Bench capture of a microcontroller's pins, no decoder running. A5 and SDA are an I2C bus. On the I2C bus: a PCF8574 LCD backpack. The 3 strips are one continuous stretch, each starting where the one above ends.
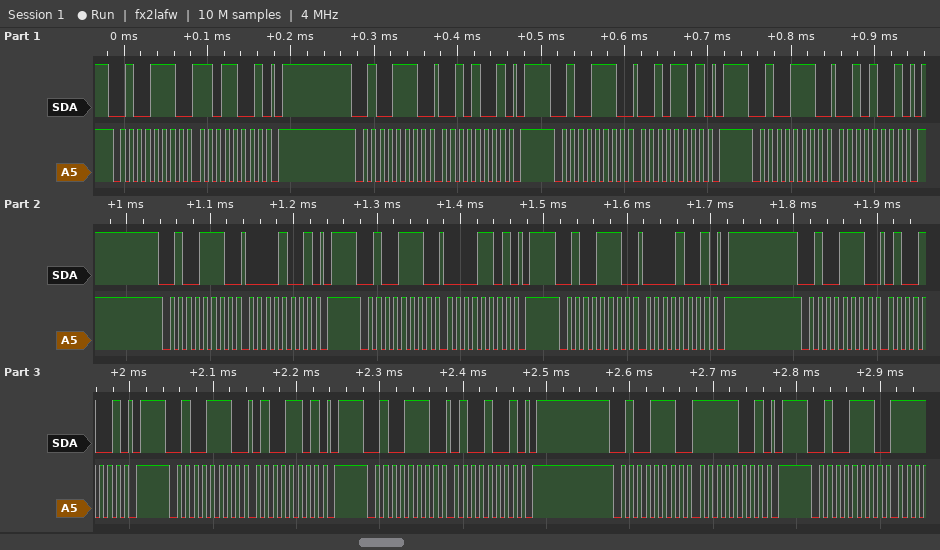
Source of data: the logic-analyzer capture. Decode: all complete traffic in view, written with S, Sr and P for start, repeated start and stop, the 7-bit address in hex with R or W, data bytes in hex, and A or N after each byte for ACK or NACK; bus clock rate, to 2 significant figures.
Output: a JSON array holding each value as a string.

["S 27W A D9 A P S 27W A 29 A P S 27W A 2D A P S 27W A 29 A P S 27W A 09 A P S 27W A 0D A P S 27W A 09 A P S 27W A 49 A P S 27W A 4D A P S 27W A 49 A P S 27W A F9 A P S 27W A", "100 kHz"]
